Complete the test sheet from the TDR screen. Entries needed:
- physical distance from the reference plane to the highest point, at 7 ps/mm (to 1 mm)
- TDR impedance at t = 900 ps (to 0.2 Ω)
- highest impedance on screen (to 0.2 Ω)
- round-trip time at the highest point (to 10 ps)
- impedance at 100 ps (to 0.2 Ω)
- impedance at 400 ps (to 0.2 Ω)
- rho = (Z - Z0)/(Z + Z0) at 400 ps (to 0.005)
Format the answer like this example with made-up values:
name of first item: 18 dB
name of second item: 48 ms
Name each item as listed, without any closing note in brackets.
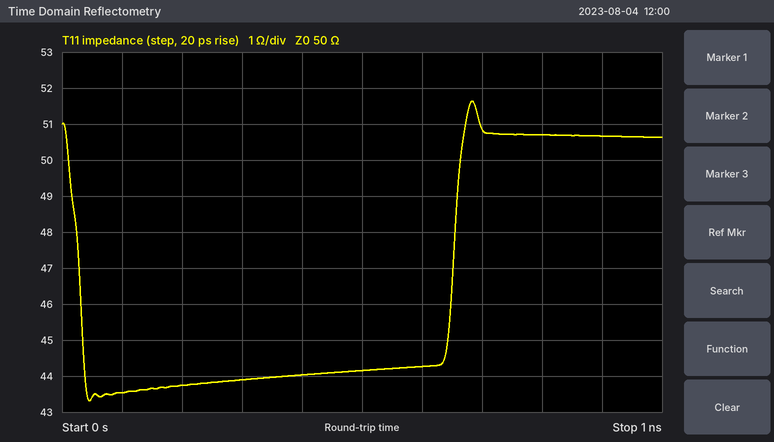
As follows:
physical distance from the reference plane to the highest point, at 7 ps/mm: 49 mm
TDR impedance at t = 900 ps: 50.6 Ω
highest impedance on screen: 51.6 Ω
round-trip time at the highest point: 680 ps
impedance at 100 ps: 43.6 Ω
impedance at 400 ps: 44.0 Ω
rho = (Z - Z0)/(Z + Z0) at 400 ps: -0.065
